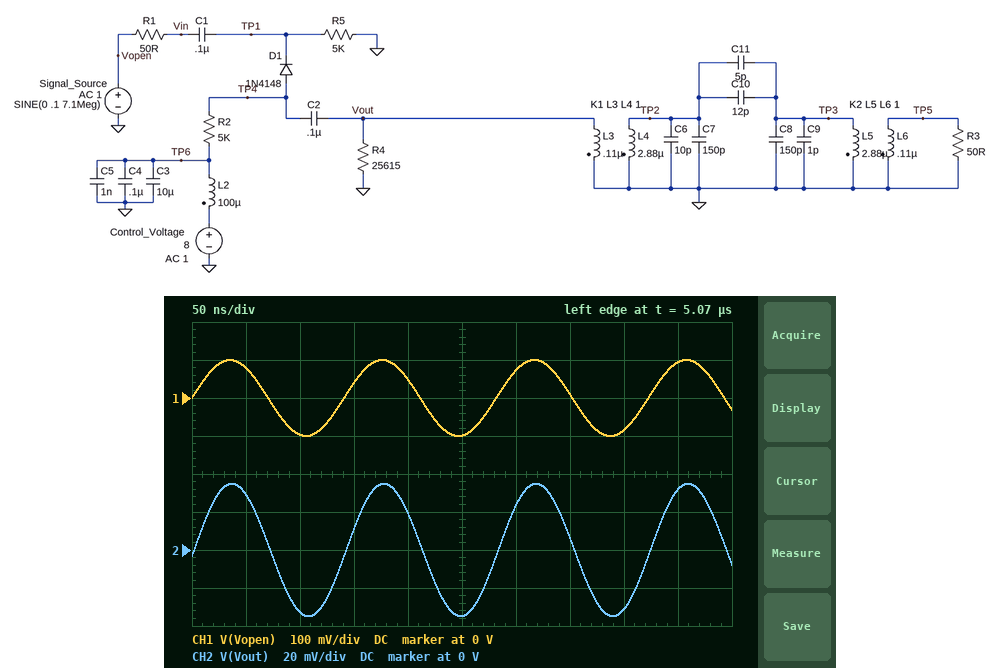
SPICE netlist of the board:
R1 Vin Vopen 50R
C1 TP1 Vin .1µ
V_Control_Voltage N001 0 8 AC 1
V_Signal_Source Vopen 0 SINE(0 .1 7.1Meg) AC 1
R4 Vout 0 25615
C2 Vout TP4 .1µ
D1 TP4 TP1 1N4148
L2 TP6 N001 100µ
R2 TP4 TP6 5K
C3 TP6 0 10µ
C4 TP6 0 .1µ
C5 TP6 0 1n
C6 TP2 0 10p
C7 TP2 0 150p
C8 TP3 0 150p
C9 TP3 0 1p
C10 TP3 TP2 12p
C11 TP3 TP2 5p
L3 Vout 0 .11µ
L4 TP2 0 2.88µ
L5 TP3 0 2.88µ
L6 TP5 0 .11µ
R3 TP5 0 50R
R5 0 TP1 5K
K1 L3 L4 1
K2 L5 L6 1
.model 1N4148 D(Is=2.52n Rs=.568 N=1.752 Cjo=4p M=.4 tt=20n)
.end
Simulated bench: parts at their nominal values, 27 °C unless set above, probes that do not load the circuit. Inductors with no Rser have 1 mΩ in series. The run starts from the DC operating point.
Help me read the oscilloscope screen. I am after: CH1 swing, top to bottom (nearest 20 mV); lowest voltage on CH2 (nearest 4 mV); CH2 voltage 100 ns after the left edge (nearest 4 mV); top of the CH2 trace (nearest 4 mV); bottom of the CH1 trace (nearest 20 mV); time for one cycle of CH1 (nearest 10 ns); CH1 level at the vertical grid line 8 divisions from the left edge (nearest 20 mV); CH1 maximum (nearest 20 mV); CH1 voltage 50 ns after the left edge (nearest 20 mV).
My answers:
200 mV
-36 mV
-32 mV
36 mV
-100 mV
140 ns
-80 mV
100 mV
80 mV
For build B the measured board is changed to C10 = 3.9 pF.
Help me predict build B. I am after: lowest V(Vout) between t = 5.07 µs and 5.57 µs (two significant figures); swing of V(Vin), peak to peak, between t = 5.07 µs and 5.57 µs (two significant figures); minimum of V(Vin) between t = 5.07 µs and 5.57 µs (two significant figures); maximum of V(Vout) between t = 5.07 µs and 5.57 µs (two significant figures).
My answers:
-80 mV
160 mV
-82 mV
80 mV
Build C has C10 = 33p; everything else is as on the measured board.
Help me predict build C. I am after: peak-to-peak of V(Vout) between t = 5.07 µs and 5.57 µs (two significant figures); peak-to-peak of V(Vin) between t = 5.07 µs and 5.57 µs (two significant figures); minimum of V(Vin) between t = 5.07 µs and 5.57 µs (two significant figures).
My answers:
30 mV
120 mV
-48 mV
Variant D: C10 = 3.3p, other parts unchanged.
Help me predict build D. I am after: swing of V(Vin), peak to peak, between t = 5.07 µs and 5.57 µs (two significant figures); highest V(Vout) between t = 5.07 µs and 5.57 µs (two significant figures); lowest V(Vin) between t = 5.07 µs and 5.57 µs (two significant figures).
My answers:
160 mV
82 mV
-82 mV
